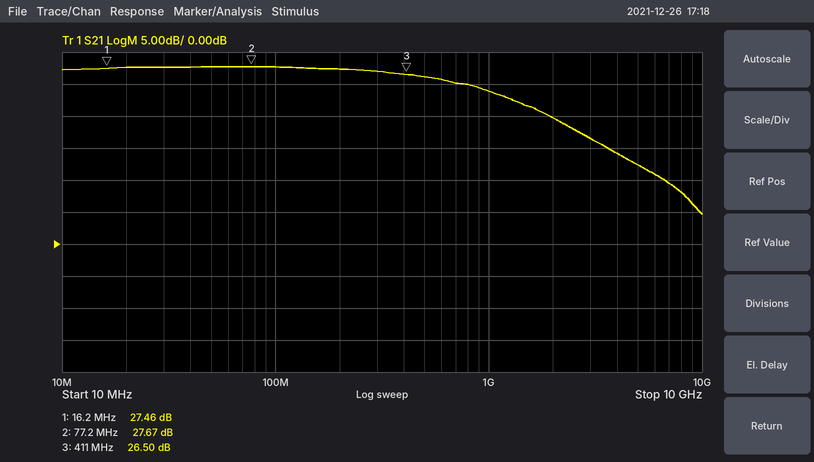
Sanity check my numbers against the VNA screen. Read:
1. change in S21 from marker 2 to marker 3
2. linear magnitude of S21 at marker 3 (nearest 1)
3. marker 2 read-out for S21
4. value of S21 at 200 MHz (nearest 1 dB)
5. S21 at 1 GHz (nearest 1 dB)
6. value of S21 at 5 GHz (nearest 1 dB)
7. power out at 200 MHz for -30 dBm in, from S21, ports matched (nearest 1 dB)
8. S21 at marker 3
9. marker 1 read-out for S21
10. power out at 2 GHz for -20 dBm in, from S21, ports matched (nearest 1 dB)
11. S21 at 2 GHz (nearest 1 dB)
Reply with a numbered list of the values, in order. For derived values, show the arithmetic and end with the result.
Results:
1. 26.5 − (27.67) = -1.17 dB
2. 10^(26.5/20) ≈ 21
3. 27.67 dB
4. 27 dB
5. 24 dB
6. 12 dB
7. -30 dBm + (27 dB) = -3 dBm
8. 26.50 dB
9. 27.46 dB
10. -20 dBm + (20 dB) = 0 dBm
11. 20 dB
